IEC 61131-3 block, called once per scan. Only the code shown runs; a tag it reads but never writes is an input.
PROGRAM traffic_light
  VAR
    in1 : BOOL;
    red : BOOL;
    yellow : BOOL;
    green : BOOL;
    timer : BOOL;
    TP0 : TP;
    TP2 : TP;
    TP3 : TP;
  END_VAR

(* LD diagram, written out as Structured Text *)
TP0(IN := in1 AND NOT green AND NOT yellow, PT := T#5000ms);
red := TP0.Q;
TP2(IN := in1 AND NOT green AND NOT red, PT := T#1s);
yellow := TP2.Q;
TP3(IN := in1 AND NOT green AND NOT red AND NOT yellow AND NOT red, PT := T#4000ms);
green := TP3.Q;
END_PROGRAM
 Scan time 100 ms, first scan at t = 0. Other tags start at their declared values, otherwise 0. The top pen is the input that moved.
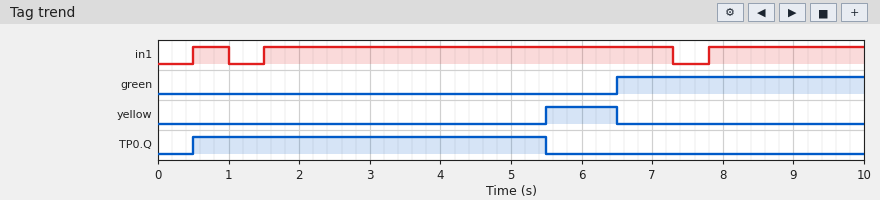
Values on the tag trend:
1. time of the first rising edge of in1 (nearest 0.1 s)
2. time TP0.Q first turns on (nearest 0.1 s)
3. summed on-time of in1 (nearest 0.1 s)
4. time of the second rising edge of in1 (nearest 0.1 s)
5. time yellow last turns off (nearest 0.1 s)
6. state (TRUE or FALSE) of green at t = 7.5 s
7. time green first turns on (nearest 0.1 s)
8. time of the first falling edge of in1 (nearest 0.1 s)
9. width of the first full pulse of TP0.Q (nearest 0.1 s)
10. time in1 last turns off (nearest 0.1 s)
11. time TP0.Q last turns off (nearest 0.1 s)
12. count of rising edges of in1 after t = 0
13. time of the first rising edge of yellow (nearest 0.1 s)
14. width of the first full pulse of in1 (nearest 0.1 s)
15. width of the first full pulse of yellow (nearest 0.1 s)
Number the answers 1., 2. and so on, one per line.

1. 0.5 s
2. 0.5 s
3. 8.5 s
4. 1.5 s
5. 6.5 s
6. TRUE
7. 6.5 s
8. 1.0 s
9. 5.0 s
10. 7.3 s
11. 5.5 s
12. 3
13. 5.5 s
14. 0.5 s
15. 1.0 s
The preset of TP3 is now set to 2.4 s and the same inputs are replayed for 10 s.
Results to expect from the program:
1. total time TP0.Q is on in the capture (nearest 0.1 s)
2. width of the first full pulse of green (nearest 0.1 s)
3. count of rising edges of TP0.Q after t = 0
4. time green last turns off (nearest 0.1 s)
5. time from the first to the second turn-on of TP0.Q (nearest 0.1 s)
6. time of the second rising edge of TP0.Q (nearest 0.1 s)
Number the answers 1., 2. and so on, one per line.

1. 6.0 s
2. 2.4 s
3. 2
4. 8.9 s
5. 8.5 s
6. 9.0 s
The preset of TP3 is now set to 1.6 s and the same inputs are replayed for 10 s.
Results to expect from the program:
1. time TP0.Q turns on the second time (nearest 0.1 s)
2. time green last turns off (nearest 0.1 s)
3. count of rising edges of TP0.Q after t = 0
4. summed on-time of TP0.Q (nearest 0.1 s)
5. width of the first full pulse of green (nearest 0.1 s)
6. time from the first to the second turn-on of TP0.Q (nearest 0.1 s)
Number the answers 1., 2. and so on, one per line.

1. 8.2 s
2. 8.1 s
3. 2
4. 6.8 s
5. 1.6 s
6. 7.7 s
